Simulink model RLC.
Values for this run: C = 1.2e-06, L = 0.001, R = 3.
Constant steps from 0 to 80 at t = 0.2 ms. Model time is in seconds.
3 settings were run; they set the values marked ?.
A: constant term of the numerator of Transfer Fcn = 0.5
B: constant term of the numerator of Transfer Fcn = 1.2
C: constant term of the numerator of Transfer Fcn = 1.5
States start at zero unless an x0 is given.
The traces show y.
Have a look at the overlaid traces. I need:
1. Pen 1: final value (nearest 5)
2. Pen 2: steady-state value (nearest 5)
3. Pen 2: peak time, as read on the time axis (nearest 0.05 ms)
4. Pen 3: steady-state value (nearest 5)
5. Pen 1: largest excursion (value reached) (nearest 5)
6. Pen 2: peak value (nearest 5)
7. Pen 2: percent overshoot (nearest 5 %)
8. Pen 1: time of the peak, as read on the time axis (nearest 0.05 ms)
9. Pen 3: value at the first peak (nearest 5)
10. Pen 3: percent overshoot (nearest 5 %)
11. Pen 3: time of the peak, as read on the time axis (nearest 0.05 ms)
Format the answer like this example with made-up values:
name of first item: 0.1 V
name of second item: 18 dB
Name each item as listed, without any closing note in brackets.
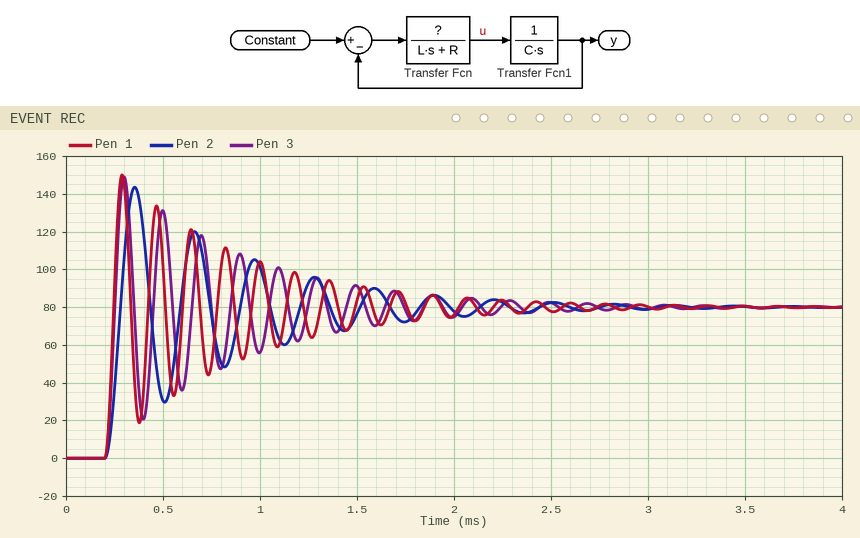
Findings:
Pen 1: final value: 80
Pen 2: steady-state value: 80
Pen 2: peak time, as read on the time axis: 0.35 ms
Pen 3: steady-state value: 80
Pen 1: largest excursion (value reached): 150
Pen 2: peak value: 145
Pen 2: percent overshoot: 80 %
Pen 1: time of the peak, as read on the time axis: 0.30 ms
Pen 3: value at the first peak: 150
Pen 3: percent overshoot: 85 %
Pen 3: time of the peak, as read on the time axis: 0.30 ms
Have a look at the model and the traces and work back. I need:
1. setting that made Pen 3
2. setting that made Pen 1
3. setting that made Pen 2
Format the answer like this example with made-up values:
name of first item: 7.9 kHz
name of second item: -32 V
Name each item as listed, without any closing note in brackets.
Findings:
setting that made Pen 3: B
setting that made Pen 1: C
setting that made Pen 2: A
